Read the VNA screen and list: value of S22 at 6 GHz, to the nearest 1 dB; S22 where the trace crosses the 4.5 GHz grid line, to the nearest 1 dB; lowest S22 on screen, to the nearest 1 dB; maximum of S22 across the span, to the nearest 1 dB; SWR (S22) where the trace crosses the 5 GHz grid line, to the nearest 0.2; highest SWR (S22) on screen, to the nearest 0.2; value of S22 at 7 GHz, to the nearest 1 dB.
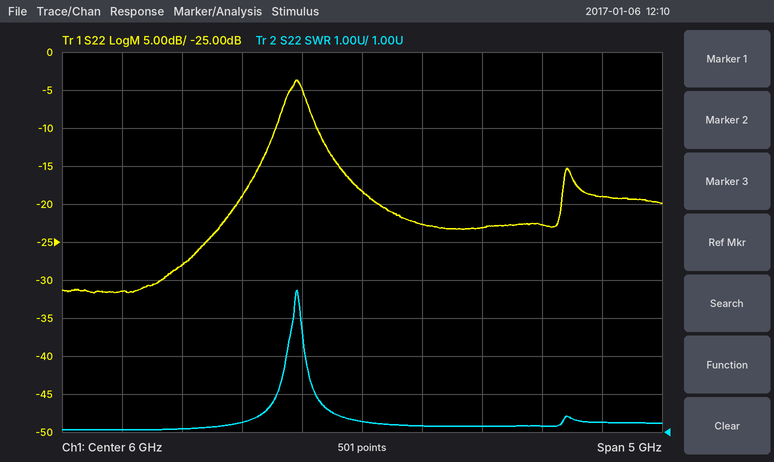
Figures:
-18 dB
-28 dB
-32 dB
-4 dB
1.2
4.8
-23 dB
